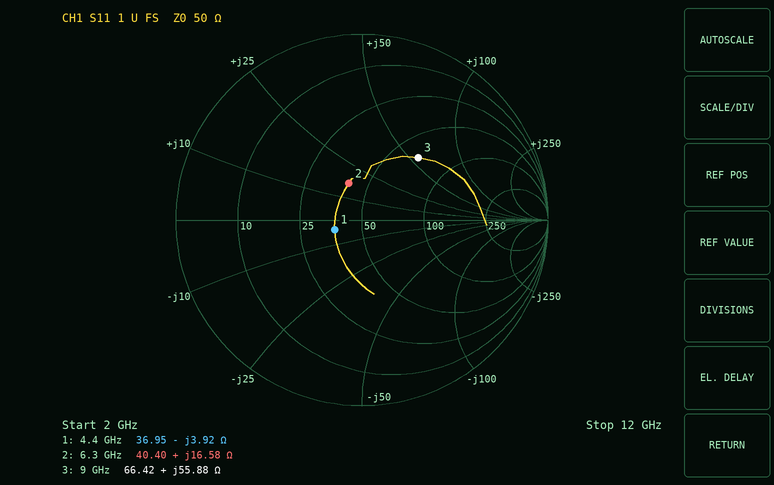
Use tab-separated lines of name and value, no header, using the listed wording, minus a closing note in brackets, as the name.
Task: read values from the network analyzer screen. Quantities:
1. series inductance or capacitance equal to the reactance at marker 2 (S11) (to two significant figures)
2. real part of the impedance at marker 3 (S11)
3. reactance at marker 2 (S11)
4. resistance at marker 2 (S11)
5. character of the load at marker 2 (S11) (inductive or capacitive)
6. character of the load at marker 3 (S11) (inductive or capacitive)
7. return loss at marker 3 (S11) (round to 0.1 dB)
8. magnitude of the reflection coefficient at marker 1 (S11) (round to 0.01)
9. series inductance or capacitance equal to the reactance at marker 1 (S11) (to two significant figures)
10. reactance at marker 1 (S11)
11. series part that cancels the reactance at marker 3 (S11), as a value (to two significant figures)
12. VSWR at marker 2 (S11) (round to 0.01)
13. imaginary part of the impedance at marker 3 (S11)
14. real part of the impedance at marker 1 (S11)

series inductance or capacitance equal to the reactance at marker 2 (S11)	420 pH
real part of the impedance at marker 3	66.42 Ω
reactance at marker 2	+16.58 Ω
resistance at marker 2	40.40 Ω
character of the load at marker 2 (S11)	inductive
character of the load at marker 3 (S11)	inductive
return loss at marker 3 (S11)	6.9 dB
magnitude of the reflection coefficient at marker 1 (S11)	0.16
series inductance or capacitance equal to the reactance at marker 1 (S11)	9.2 pF
reactance at marker 1	-3.92 Ω
series part that cancels the reactance at marker 3 (S11), as a value	320 fF
VSWR at marker 2 (S11)	1.53
imaginary part of the impedance at marker 3	+55.88 Ω
real part of the impedance at marker 1	36.95 Ω
